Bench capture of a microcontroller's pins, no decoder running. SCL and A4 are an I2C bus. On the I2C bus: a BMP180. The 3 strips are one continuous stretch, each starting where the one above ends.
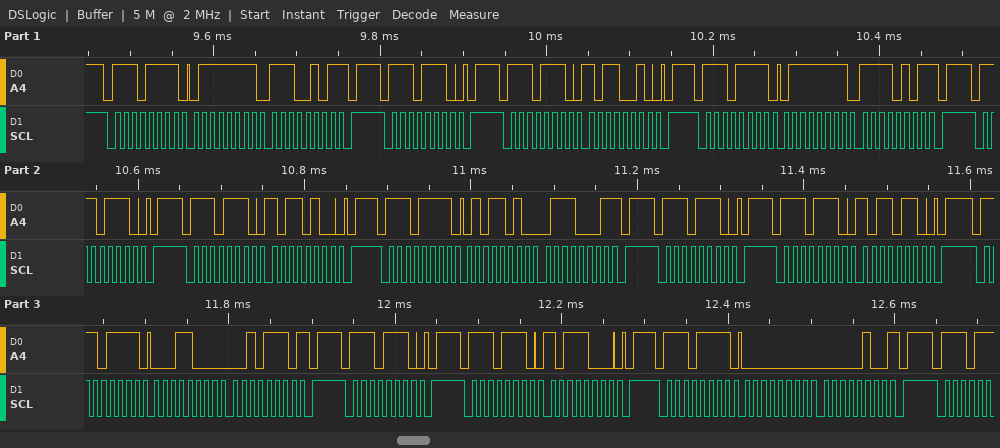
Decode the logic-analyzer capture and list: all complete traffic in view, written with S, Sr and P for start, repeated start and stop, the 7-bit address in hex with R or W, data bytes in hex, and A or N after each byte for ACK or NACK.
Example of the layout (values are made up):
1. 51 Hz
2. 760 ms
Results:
1. S 77R A 7F A E5 N P S 77W A P S 77W A B2 A P S 77R A 7F A F5 N P S 77W A P S 77W A B4 A P S 77R A 5A A 71 N P S 77W A P S 77W A B6 A P S 77R A 18 A 2E N P S 77W A P S 77W A B8 A P S 77R A 00 A 04 N P
